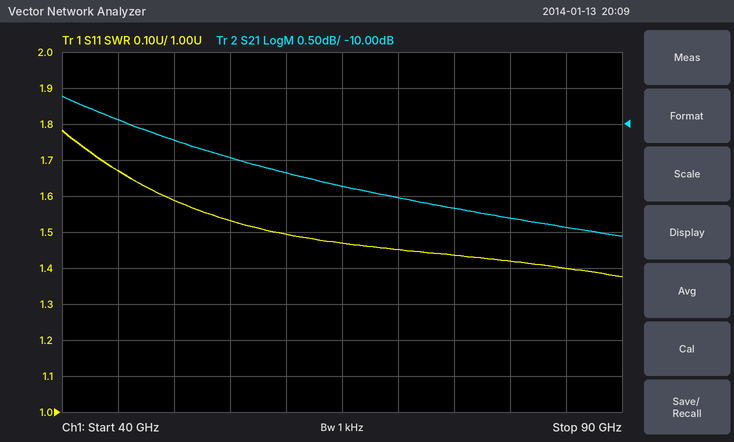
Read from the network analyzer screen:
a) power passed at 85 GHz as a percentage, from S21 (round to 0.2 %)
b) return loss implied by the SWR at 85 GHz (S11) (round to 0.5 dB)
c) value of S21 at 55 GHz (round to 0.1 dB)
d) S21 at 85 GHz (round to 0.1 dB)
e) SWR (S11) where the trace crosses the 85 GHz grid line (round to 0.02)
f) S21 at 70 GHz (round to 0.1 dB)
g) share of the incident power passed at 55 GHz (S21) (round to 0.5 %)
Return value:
7.2 %
15.5 dB
-10.5 dB
-11.4 dB
1.40
-11.0 dB
9.0 %
